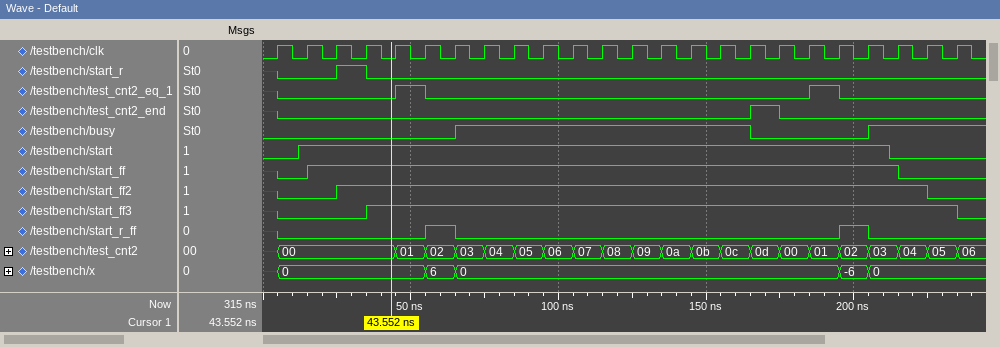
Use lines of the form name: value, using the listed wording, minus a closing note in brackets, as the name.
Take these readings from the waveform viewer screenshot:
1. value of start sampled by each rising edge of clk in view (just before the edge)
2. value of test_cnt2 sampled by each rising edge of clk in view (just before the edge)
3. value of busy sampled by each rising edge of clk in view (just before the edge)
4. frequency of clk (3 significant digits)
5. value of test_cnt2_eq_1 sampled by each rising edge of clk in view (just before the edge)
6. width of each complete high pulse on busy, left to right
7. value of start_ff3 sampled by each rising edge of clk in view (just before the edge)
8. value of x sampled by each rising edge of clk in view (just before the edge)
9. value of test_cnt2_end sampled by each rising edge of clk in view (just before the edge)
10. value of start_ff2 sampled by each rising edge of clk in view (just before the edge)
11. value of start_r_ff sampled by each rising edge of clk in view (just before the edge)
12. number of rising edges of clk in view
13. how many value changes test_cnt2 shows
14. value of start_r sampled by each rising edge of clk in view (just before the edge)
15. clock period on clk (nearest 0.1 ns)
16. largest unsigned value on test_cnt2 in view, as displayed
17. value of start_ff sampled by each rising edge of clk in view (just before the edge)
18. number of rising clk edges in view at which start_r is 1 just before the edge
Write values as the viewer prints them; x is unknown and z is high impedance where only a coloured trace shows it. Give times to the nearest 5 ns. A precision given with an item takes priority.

value of start sampled by each rising edge of clk in view: 0 1 1 1 1 1 1 1 1 1 1 1 1 1 1 1 1 1 1 1 1 0 0 0
value of test_cnt2 sampled by each rising edge of clk in view: x, 00, 00, 00, 00, 01, 02, 03, 04, 05, 06, 07, 08, 09, 0a, 0b, 0c, 0d, 00, 01, 02, 03, 04, 05
value of busy sampled by each rising edge of clk in view: 0 0 0 0 0 0 0 1 1 1 1 1 1 1 1 1 1 0 0 0 0 1 1 1
frequency of clk: 100 MHz
value of test_cnt2_eq_1 sampled by each rising edge of clk in view: x 0 0 0 0 1 0 0 0 0 0 0 0 0 0 0 0 0 0 1 0 0 0 0
width of each complete high pulse on busy, left to right: 100 ns
value of start_ff3 sampled by each rising edge of clk in view: x 0 0 0 1 1 1 1 1 1 1 1 1 1 1 1 1 1 1 1 1 1 1 1
value of x sampled by each rising edge of clk in view: x, 0, 0, 0, 0, 0, 6, 0, 0, 0, 0, 0, 0, 0, 0, 0, 0, 0, 0, 0, -6, 0, 0, 0
value of test_cnt2_end sampled by each rising edge of clk in view: x 0 0 0 0 0 0 0 0 0 0 0 0 0 0 0 0 1 0 0 0 0 0 0
value of start_ff2 sampled by each rising edge of clk in view: x 0 0 1 1 1 1 1 1 1 1 1 1 1 1 1 1 1 1 1 1 1 1 0
value of start_r_ff sampled by each rising edge of clk in view: x 0 0 0 0 0 1 0 0 0 0 0 0 0 0 0 0 0 0 0 1 0 0 0
number of rising edges of clk in view: 24
how many value changes test_cnt2 shows: 21
value of start_r sampled by each rising edge of clk in view: x 0 0 1 0 0 0 0 0 0 0 0 0 0 0 0 0 0 0 0 0 0 0 0
clock period on clk: 10 ns
largest unsigned value on test_cnt2 in view, as displayed: 0d
value of start_ff sampled by each rising edge of clk in view: x 0 1 1 1 1 1 1 1 1 1 1 1 1 1 1 1 1 1 1 1 1 0 0
number of rising clk edges in view at which start_r is 1 just before the edge: 1
